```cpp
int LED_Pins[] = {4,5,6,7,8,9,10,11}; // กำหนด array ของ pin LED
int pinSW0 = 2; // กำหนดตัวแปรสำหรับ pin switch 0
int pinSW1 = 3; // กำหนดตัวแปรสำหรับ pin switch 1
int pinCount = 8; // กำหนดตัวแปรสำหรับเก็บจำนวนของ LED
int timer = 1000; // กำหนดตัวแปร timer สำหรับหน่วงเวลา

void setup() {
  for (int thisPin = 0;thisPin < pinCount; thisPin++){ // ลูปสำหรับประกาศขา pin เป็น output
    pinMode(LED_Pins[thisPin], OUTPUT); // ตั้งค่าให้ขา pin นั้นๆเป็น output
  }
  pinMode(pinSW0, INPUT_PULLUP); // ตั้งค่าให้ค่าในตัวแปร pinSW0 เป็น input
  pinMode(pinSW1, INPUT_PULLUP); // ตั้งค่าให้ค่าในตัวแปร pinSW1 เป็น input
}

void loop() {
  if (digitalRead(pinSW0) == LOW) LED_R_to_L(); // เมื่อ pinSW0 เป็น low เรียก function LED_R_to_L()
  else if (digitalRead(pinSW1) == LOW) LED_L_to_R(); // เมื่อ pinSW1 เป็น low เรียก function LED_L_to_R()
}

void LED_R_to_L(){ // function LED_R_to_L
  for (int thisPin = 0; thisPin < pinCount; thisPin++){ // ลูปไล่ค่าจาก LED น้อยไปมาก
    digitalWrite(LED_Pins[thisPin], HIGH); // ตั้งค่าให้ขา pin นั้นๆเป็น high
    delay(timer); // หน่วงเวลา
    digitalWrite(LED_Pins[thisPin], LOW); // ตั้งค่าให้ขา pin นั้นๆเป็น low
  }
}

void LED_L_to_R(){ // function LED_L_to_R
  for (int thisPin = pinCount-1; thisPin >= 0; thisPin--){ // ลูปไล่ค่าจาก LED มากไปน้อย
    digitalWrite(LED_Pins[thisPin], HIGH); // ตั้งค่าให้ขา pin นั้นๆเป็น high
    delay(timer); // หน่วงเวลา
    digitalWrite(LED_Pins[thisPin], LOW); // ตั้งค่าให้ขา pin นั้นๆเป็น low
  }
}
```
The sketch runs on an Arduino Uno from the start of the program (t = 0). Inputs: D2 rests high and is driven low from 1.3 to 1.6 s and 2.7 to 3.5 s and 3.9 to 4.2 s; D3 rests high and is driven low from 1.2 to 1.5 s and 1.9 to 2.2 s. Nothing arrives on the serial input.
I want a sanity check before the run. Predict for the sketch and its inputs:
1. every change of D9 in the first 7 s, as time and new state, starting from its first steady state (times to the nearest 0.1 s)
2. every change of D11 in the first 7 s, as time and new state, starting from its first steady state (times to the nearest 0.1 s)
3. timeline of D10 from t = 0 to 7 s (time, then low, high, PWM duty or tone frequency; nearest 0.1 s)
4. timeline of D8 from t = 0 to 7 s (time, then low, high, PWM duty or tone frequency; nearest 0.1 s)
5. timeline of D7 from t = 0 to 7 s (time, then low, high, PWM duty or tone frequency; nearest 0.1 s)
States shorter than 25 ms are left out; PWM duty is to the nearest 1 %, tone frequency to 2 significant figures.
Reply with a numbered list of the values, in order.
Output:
1. 0 s low; 3.2 s high; 4.2 s low
2. 0 s low; 1.2 s high; 2.2 s low
3. 0 s low; 2.2 s high; 3.2 s low
4. 0 s low; 4.2 s high; 5.2 s low
5. 0 s low; 5.2 s high; 6.2 s low
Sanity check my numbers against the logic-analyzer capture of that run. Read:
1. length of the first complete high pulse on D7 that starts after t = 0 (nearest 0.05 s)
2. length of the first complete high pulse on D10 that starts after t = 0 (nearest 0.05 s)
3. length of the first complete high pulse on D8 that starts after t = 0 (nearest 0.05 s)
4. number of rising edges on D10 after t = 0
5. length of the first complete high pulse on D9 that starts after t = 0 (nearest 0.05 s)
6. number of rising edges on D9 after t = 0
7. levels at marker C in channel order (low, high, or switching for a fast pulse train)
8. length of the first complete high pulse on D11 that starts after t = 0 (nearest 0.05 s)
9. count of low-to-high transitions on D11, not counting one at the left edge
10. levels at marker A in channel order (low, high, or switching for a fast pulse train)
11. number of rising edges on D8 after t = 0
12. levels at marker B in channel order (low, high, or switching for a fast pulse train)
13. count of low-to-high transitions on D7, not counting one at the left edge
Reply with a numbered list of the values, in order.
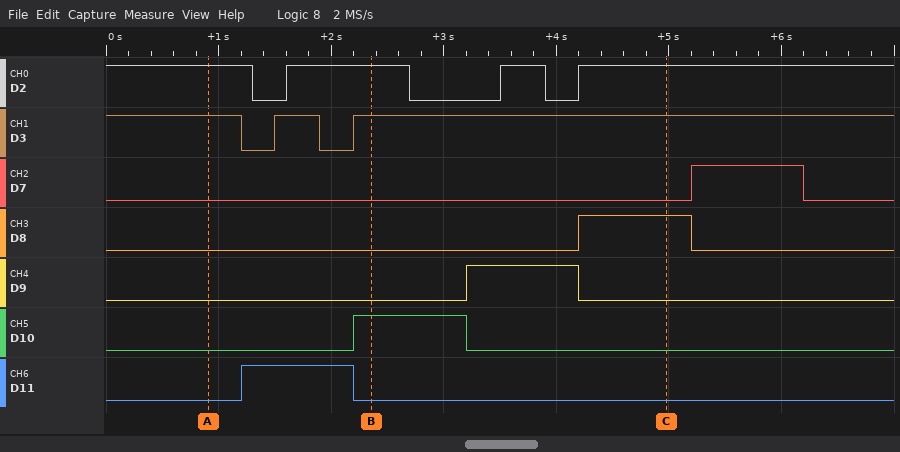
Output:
1. 1.00 s
2. 1.00 s
3. 1.00 s
4. 1
5. 1.00 s
6. 1
7. D2 high, D3 high, D7 low, D8 high, D9 low, D10 low, D11 low
8. 1.00 s
9. 1
10. D2 high, D3 high, D7 low, D8 low, D9 low, D10 low, D11 low
11. 1
12. D2 high, D3 high, D7 low, D8 low, D9 low, D10 high, D11 low
13. 1
